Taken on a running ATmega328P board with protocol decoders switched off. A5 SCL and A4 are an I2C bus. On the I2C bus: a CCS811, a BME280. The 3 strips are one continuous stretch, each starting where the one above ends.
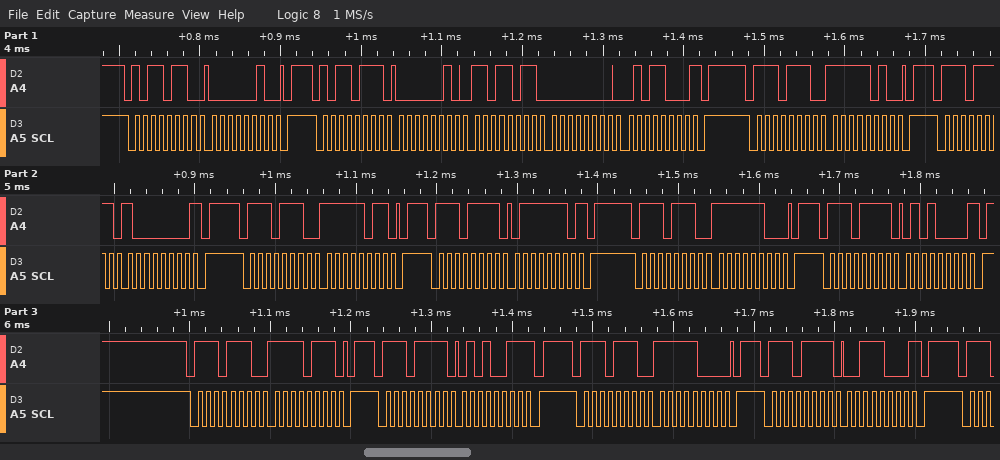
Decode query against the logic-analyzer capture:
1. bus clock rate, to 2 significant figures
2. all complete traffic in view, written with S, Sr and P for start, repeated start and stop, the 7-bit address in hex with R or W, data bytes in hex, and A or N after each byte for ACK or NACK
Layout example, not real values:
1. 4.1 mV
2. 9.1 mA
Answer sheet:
1. 100 kHz
2. S 5BW A 02 A P S 5BR A 02 A DB A 00 A 58 N P S 77W A FA A P S 77R A 80 N P S 77W A FB A P S 77R A 7E N P S 77W A FC A P S 77R A 50 N P S 77W A F7 A P S 77R A 53 N P S 77W A F8 A P S 77R A 38 N P
